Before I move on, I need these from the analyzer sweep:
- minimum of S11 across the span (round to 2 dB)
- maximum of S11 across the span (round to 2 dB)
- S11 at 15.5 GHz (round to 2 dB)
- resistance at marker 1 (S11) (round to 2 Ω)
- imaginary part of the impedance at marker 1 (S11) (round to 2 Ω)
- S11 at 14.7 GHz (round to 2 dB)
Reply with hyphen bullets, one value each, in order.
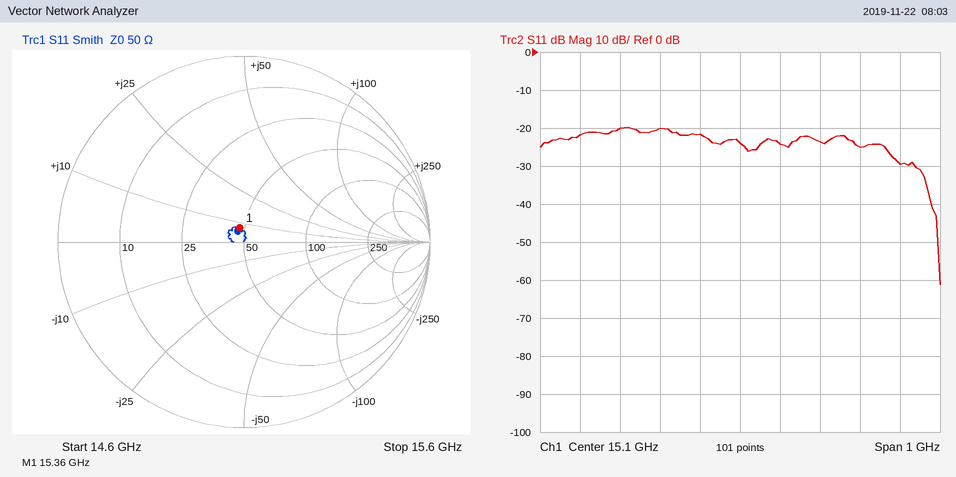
- -62 dB
- -20 dB
- -30 dB
- 48 Ω
- +8 Ω
- -22 dB
